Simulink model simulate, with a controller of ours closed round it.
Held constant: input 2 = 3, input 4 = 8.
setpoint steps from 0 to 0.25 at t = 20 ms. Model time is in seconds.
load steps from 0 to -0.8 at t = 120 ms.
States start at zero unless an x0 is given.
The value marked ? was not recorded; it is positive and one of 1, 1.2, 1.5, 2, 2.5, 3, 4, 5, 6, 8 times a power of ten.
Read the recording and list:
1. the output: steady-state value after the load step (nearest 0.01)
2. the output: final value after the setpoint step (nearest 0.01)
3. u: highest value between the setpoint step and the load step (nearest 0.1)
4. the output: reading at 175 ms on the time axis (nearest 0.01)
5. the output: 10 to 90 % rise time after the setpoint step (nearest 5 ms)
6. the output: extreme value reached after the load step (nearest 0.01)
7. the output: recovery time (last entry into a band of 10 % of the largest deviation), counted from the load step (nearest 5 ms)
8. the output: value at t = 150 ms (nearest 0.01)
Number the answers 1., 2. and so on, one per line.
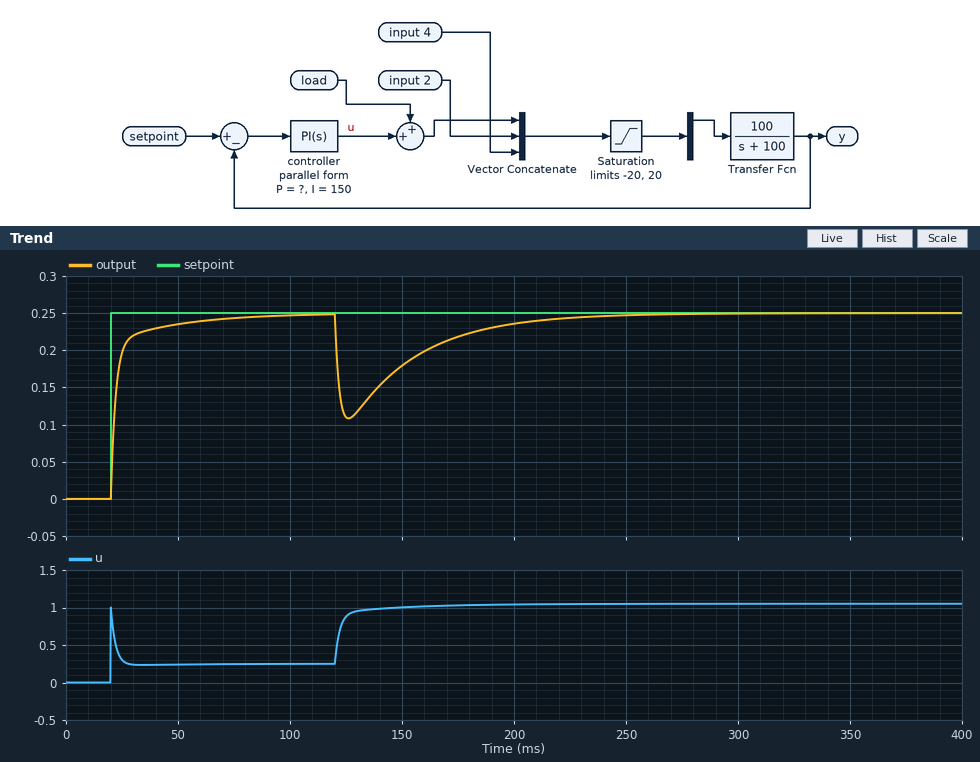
1. 0.25
2. 0.25
3. 1.0
4. 0.22
5. 15 ms
6. 0.11
7. 80 ms
8. 0.18
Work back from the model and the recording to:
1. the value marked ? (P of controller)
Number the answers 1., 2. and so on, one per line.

1. 4
